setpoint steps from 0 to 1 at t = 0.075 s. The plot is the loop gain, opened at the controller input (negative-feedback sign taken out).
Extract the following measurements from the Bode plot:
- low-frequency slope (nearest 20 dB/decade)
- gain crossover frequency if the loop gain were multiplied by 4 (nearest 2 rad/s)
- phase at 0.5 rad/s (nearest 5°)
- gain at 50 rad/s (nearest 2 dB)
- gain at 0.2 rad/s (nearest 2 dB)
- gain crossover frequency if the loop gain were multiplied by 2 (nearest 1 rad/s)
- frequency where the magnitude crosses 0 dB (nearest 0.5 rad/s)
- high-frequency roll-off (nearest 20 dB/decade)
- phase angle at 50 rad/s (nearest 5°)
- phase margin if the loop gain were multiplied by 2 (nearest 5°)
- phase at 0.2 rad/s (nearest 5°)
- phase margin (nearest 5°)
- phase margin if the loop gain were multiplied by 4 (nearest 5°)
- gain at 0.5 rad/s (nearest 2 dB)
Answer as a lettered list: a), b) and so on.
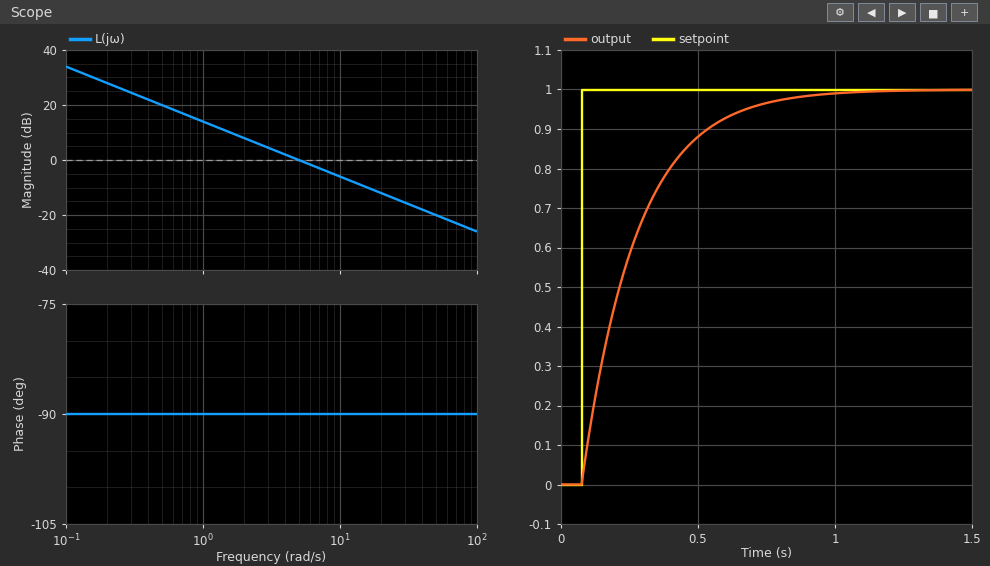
a) -20 dB/decade
b) 20 rad/s
c) -90°
d) -20 dB
e) 28 dB
f) 10 rad/s
g) 5.0 rad/s
h) -20 dB/decade
i) -90°
j) 90°
k) -90°
l) 90°
m) 90°
n) 20 dB
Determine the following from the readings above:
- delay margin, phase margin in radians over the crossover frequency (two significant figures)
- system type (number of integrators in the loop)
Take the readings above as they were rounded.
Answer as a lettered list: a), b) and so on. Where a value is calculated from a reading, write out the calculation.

a) 90 × π / 180 / 5 = 0.31 s
b) 1
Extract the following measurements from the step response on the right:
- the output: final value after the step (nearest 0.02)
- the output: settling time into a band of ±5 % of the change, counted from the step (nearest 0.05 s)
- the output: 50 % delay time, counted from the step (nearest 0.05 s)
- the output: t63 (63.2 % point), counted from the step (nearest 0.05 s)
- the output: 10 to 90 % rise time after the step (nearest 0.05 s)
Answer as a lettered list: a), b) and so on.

a) 1.00
b) 0.60 s
c) 0.15 s
d) 0.20 s
e) 0.45 s
